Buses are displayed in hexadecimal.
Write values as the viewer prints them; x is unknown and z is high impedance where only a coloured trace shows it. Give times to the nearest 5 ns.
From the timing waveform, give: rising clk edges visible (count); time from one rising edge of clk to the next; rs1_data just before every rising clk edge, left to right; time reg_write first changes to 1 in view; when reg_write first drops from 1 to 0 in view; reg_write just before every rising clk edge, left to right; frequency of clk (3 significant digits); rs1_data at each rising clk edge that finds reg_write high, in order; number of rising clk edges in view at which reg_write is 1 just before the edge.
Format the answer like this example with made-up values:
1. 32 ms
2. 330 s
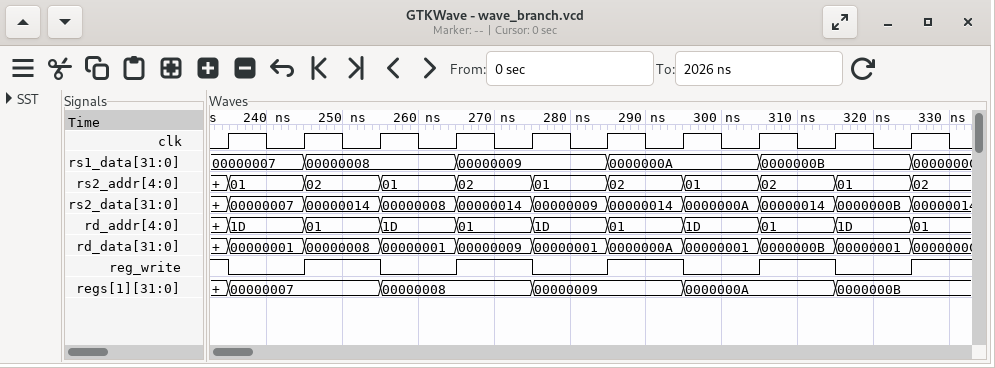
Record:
1. 10
2. 10 ns
3. 00000007, 00000007, 00000008, 00000008, 00000009, 00000009, 0000000A, 0000000A, 0000000B, 0000000B
4. 245 ns
5. 235 ns
6. 1 0 1 0 1 0 1 0 1 0
7. 100 MHz
8. 00000007, 00000008, 00000009, 0000000A, 0000000B
9. 5
